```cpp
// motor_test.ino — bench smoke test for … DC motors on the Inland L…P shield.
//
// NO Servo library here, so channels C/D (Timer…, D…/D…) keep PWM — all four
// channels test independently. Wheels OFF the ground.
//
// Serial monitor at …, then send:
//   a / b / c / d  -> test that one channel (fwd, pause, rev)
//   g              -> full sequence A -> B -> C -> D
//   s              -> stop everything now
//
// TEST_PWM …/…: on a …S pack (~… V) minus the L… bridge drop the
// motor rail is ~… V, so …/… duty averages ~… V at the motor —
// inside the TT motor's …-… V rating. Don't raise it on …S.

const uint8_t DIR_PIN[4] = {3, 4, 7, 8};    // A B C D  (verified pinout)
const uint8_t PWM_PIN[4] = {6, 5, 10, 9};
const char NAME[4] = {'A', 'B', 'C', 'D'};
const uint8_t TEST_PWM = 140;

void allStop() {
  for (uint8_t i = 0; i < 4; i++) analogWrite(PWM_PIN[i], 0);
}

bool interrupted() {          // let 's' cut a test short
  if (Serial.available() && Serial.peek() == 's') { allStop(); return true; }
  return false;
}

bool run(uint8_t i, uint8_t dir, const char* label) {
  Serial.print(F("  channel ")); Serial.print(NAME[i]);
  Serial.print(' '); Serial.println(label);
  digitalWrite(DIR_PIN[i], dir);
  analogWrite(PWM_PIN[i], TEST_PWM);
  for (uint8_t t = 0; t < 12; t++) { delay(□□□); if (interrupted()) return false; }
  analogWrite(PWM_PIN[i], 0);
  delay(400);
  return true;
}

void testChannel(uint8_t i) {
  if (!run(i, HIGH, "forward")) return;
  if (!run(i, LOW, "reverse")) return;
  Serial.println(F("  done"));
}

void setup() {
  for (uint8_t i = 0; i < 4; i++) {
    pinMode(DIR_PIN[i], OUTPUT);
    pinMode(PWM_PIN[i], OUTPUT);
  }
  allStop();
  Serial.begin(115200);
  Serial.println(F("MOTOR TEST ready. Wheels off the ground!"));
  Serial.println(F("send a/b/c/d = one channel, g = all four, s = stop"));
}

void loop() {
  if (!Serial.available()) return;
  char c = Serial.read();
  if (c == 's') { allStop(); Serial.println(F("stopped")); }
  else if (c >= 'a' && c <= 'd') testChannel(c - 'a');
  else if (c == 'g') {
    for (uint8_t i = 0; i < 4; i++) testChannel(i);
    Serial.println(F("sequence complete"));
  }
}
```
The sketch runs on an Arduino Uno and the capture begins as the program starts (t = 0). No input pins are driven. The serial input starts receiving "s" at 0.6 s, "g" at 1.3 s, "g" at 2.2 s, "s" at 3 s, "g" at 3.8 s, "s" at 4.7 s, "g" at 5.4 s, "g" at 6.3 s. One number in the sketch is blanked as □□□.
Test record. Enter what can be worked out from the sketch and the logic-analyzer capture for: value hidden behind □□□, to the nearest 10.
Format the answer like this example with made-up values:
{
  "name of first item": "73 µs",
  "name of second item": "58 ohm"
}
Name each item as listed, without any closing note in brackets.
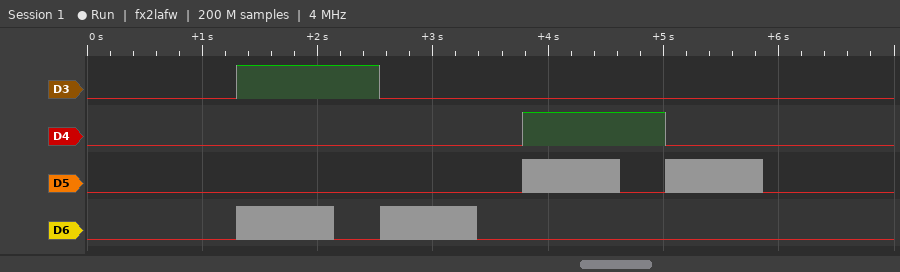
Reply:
{
  "value hidden behind □□□, to the nearest 10": "70"
}
